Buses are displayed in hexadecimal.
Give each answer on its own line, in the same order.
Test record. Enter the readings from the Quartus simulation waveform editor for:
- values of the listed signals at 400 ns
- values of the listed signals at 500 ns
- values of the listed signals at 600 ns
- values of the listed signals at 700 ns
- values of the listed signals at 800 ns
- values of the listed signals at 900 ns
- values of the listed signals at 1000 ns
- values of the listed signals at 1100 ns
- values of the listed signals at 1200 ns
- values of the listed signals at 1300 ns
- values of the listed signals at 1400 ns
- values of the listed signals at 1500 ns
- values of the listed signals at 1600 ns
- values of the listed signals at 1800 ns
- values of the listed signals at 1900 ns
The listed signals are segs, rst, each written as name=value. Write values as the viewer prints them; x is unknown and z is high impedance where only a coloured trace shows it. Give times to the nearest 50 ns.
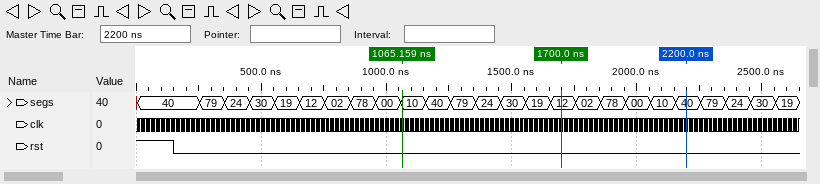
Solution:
segs=24, rst=0
segs=30, rst=0
segs=19, rst=0
segs=12, rst=0
segs=02, rst=0
segs=78, rst=0
segs=00, rst=0
segs=10, rst=0
segs=40, rst=0
segs=79, rst=0
segs=24, rst=0
segs=30, rst=0
segs=19, rst=0
segs=02, rst=0
segs=78, rst=0
